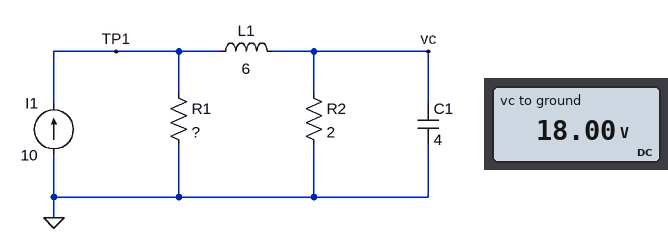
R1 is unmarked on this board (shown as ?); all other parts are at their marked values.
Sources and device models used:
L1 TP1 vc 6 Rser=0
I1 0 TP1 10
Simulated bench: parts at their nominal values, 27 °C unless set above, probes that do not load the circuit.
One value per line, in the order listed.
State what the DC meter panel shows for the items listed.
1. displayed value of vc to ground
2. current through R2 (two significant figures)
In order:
18.00 V
9.0 A
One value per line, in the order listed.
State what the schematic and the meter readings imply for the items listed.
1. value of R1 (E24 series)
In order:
18 Ω
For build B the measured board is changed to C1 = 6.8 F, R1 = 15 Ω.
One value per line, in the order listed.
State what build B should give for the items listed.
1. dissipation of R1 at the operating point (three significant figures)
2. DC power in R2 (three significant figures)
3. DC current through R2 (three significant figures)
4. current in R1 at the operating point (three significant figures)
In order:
20.8 W
156 W
8.82 A
1.18 A
